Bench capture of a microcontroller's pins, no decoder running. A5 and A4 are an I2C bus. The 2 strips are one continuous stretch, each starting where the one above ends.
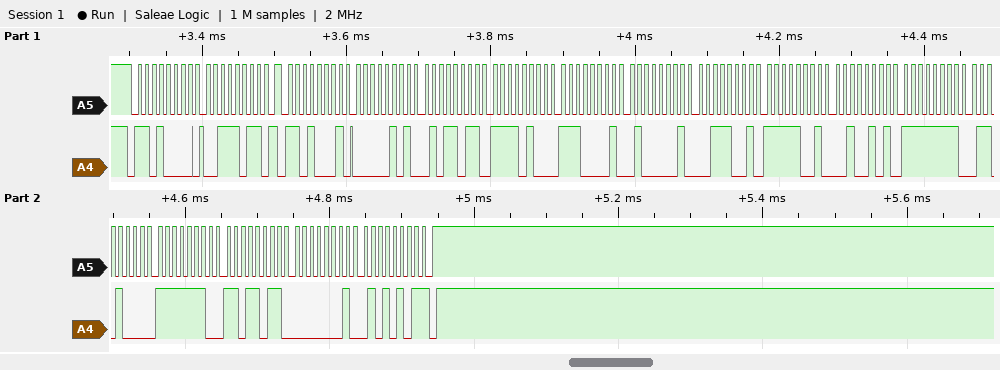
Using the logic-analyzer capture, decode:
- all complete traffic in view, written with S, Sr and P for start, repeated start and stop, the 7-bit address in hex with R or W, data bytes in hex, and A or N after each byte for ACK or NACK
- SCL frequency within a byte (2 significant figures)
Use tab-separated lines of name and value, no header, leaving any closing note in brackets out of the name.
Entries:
all complete traffic in view, written with S, Sr and P for start, repeated start and stop, the 7-bit address in hex with R or W, data bytes in hex, and A or N after each byte for ACK or NACK	S 68W A 3B A Sr 68R A 05 A 5B A F4 A E1 A 41 A 39 A F9 A 25 A FF A 68 A FE A DB A 01 A 55 N P
SCL frequency within a byte	100 kHz
